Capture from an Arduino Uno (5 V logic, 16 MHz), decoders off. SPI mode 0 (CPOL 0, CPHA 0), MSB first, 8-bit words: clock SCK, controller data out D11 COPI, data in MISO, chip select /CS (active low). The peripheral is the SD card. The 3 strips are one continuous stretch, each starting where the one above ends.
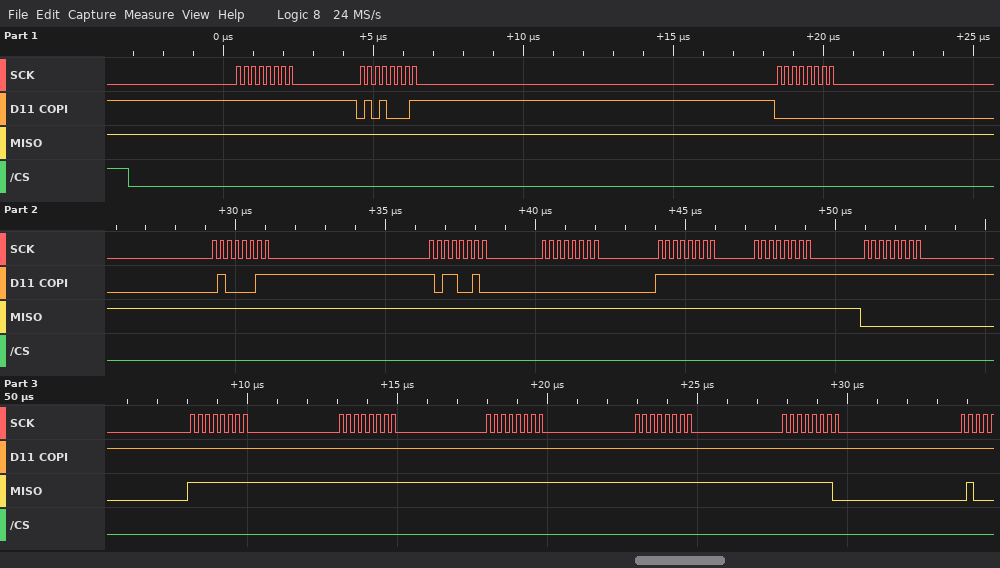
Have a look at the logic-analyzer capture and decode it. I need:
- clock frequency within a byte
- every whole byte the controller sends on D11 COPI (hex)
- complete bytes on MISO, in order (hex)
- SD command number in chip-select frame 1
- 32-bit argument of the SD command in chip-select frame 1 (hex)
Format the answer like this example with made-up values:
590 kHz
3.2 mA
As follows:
4 MHz
FF 51 00 43 B2 00 FF FF FF FF FF FF FF FF
FF FF FF FF FF FF FF FF 00 FF FF FF FF FE
CMD17
0x0043B200
